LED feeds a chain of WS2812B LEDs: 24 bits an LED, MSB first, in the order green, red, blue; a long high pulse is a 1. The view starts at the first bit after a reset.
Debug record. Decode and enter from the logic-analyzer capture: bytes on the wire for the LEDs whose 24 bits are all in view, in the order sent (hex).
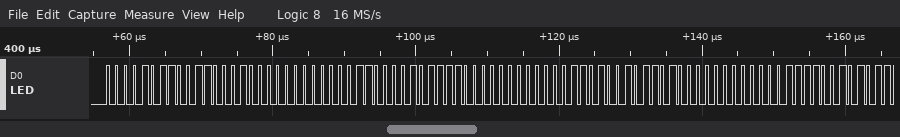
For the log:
0B 31 00 0C 2F 00 0D 2D 00
